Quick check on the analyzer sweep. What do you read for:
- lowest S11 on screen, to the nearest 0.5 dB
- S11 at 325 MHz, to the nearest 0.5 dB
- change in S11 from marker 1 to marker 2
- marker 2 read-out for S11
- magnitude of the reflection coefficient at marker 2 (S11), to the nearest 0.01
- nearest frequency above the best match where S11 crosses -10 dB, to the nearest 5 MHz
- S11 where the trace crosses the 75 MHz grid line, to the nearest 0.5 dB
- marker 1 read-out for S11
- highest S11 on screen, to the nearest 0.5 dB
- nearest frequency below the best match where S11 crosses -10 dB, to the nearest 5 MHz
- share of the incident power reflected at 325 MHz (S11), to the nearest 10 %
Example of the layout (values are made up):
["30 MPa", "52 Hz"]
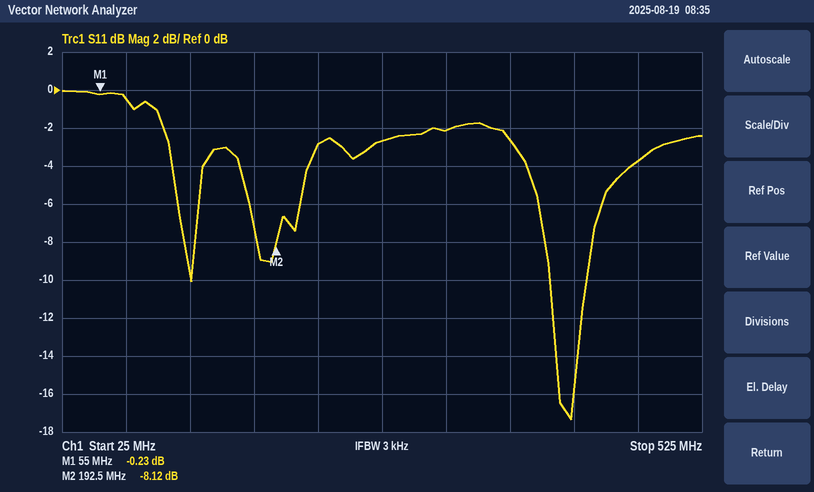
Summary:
["-17.5 dB", "-2.0 dB", "-7.89 dB", "-8.12 dB", "0.39", "435 MHz", "-0.5 dB", "-0.23 dB", "0.0 dB", "405 MHz", "60 %"]
